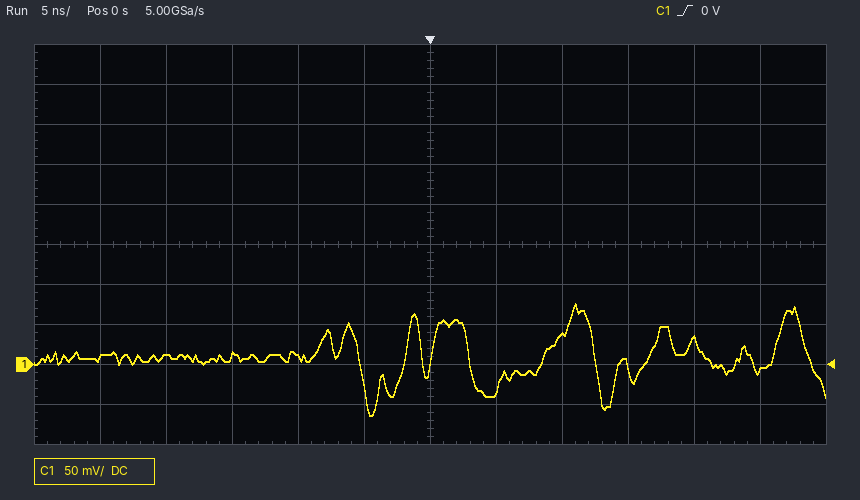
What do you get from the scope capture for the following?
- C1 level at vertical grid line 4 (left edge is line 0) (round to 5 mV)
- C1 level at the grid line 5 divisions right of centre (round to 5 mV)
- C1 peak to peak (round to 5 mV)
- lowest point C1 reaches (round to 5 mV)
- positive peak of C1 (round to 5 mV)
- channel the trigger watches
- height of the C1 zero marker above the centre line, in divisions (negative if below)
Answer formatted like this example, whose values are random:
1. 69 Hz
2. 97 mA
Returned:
1. 10 mV
2. -10 mV
3. 140 mV
4. -65 mV
5. 75 mV
6. C1
7. -3.0 div
